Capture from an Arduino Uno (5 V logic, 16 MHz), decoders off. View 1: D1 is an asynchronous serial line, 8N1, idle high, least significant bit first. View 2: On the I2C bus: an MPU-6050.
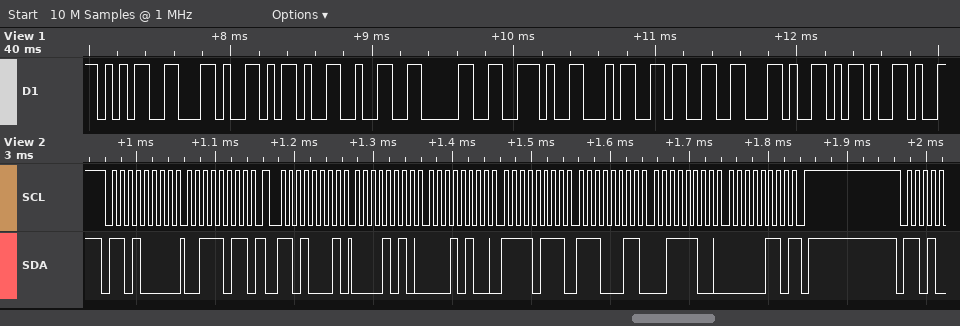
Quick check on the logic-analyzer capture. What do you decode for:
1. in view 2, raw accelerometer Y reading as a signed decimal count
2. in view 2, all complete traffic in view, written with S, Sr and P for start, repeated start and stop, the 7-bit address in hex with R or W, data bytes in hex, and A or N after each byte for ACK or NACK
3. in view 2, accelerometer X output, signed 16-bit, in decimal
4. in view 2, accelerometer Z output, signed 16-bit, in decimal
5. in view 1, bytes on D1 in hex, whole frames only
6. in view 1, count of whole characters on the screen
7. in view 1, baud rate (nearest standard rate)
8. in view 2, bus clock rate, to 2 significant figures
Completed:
-2077
S 68W A 3B A Sr 68R A 0A A 14 A F7 A E3 A 3C A 06 N P
2580
15366
35 2C 2D 32 30 2E 34 33 2C 2D
10
19200 baud
100 kHz
